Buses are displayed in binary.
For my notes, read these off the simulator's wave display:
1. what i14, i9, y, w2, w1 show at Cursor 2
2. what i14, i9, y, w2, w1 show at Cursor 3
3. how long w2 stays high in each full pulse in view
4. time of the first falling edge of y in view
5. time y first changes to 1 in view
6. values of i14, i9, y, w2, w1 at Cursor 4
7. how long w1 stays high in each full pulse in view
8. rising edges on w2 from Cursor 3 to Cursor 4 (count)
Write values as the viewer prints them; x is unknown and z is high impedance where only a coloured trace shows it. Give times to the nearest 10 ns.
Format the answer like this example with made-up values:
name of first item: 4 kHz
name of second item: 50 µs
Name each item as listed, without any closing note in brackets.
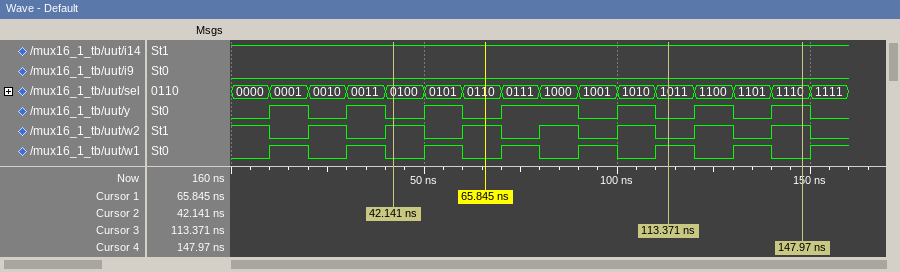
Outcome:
what i14, i9, y, w2, w1 show at Cursor 2: i14=1, i9=0, y=0, w2=1, w1=0
what i14, i9, y, w2, w1 show at Cursor 3: i14=1, i9=0, y=0, w2=0, w1=1
how long w2 stays high in each full pulse in view: 10 ns, 10 ns, 10 ns, 10 ns, 10 ns, 10 ns, 10 ns
time of the first falling edge of y in view: 20 ns
time y first changes to 1 in view: 10 ns
values of i14, i9, y, w2, w1 at Cursor 4: i14=1, i9=0, y=1, w2=1, w1=0
how long w1 stays high in each full pulse in view: 10 ns, 10 ns, 10 ns, 10 ns, 10 ns, 10 ns, 10 ns
rising edges on w2 from Cursor 3 to Cursor 4: 2
